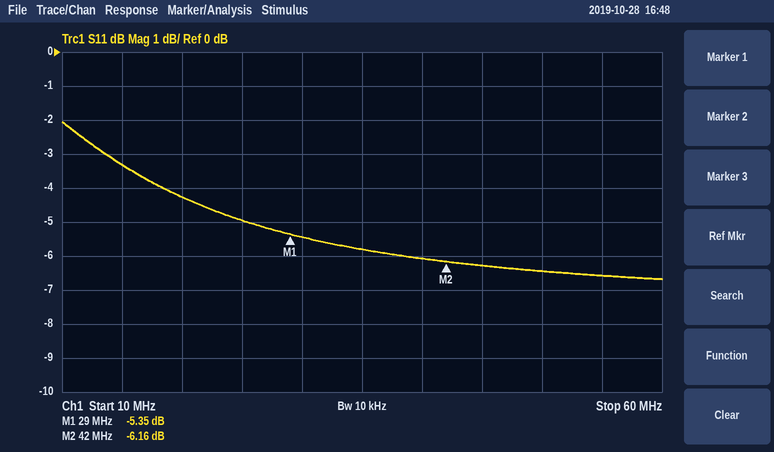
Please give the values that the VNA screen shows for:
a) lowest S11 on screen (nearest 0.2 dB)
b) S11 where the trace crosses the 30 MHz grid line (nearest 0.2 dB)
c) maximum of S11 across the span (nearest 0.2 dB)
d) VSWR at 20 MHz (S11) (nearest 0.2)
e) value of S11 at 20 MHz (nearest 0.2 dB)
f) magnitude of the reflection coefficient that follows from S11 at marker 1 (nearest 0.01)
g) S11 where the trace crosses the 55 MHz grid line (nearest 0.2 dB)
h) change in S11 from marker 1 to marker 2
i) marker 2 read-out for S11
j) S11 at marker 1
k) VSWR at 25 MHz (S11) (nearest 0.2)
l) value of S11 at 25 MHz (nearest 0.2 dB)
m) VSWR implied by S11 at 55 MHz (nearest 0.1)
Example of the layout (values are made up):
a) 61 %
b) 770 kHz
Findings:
a) -6.6 dB
b) -5.4 dB
c) -2.0 dB
d) 4.2
e) -4.2 dB
f) 0.54
g) -6.6 dB
h) -0.81 dB
i) -6.16 dB
j) -5.35 dB
k) 3.6
l) -5.0 dB
m) 2.8
